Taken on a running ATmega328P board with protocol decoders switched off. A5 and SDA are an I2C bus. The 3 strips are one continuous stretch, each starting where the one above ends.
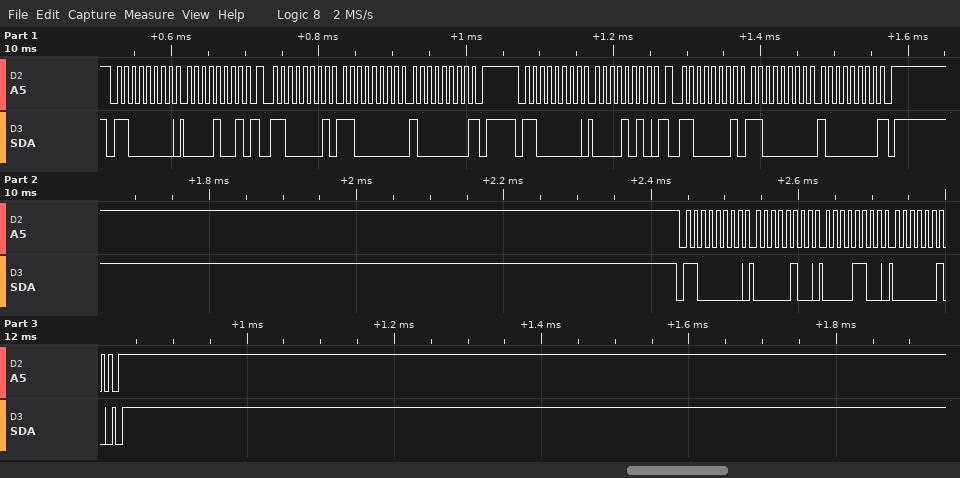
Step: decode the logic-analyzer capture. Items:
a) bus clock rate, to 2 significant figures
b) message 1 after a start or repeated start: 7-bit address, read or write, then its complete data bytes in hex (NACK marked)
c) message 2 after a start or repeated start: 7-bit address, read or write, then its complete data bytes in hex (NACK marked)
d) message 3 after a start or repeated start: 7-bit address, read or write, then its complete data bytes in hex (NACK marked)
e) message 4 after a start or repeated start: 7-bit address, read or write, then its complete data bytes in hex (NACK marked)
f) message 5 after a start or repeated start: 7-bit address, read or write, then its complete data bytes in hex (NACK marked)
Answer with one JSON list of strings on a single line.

["100 kHz", "0x60 write: 09", "0x60 read: C0 80 NACK", "0x60 write: 0A", "0x60 read: C0 80 NACK", "0x60 write: 04 0C 02"]
